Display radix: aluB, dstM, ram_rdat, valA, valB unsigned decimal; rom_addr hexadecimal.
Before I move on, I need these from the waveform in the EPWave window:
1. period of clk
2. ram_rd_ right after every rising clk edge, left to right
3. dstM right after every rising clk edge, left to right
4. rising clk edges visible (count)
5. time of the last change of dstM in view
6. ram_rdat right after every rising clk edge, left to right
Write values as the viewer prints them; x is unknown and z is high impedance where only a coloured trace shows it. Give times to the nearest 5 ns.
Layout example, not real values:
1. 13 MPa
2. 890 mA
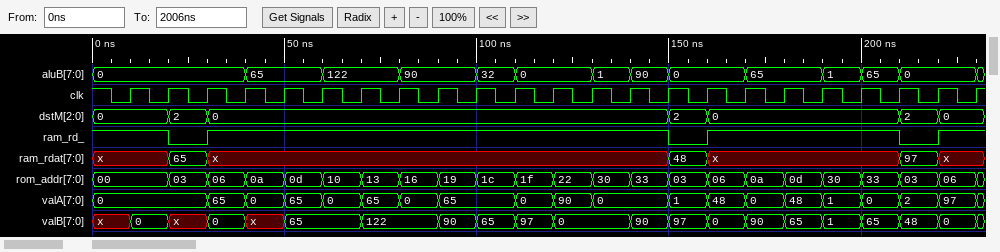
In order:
1. 10 ns
2. 1 0 1 1 1 1 1 1 1 1 1 1 1 1 0 1 1 1 1 1 0 1 1
3. 0, 2, 0, 0, 0, 0, 0, 0, 0, 0, 0, 0, 0, 0, 2, 0, 0, 0, 0, 0, 2, 0, 0
4. 23
5. 220 ns
6. x, 65, x, x, x, x, x, x, x, x, x, x, x, x, 48, x, x, x, x, x, 97, x, x
